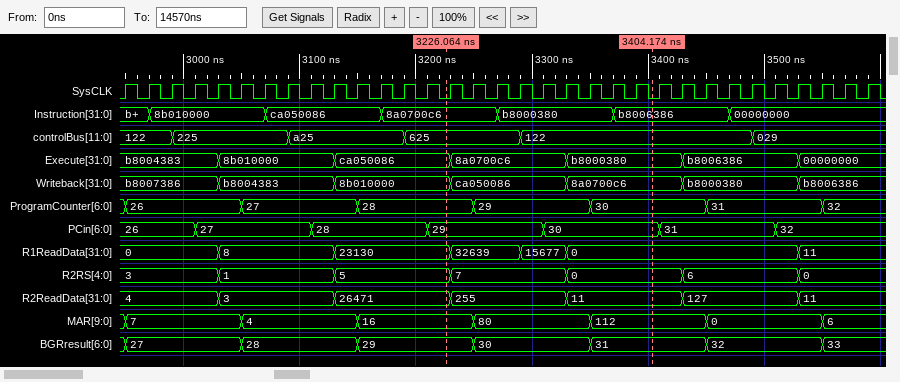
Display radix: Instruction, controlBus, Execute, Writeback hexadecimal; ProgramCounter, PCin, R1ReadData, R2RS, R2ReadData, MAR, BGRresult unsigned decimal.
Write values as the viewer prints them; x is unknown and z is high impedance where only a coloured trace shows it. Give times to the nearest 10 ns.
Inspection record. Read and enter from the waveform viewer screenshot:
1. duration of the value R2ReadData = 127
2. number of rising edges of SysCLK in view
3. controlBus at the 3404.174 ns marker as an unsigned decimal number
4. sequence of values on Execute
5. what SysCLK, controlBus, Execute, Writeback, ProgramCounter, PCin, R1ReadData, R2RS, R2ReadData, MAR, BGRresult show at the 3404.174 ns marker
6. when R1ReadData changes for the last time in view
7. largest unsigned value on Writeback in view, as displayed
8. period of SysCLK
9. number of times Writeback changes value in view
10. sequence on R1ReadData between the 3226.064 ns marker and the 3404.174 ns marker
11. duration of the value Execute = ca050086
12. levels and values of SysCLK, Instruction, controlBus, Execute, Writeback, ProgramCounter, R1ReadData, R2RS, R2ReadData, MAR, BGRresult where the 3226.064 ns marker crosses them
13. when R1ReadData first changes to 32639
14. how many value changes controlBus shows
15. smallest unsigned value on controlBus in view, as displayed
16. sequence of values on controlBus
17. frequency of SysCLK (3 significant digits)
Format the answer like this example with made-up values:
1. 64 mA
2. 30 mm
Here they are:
1. 100 ns
2. 33
3. 290
4. b8004383, 8b010000, ca050086, 8a0700c6, b8000380, b8006386, 00000000
5. SysCLK=0, controlBus=122, Execute=b8000380, Writeback=8a0700c6, ProgramCounter=30, PCin=30, R1ReadData=0, R2RS=0, R2ReadData=11, MAR=112, BGRresult=31
6. 3530 ns
7. ca050086
8. 20 ns
9. 6
10. 23130, 32639, 15677, 0
11. 100 ns
12. SysCLK=0, Instruction=8a0700c6, controlBus=625, Execute=ca050086, Writeback=8b010000, ProgramCounter=28, R1ReadData=23130, R2RS=5, R2ReadData=26471, MAR=16, BGRresult=29
13. 3230 ns
14. 5
15. 029
16. 122, 225, a25, 625, 122, 029
17. 50.0 MHz
